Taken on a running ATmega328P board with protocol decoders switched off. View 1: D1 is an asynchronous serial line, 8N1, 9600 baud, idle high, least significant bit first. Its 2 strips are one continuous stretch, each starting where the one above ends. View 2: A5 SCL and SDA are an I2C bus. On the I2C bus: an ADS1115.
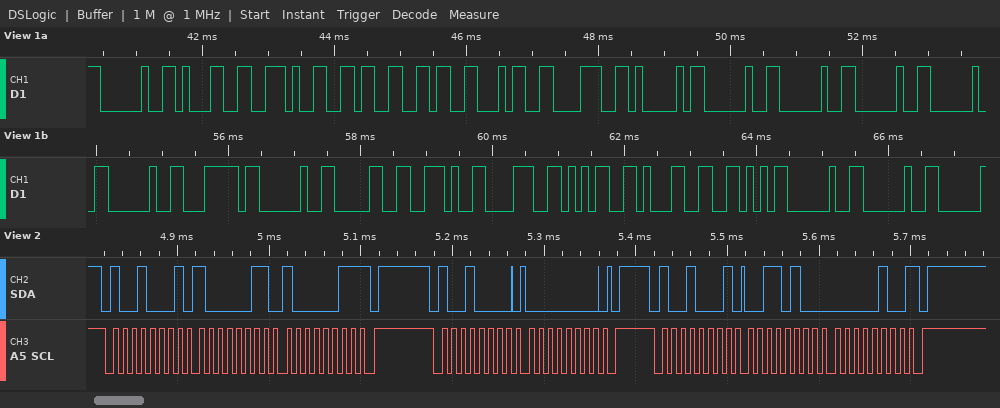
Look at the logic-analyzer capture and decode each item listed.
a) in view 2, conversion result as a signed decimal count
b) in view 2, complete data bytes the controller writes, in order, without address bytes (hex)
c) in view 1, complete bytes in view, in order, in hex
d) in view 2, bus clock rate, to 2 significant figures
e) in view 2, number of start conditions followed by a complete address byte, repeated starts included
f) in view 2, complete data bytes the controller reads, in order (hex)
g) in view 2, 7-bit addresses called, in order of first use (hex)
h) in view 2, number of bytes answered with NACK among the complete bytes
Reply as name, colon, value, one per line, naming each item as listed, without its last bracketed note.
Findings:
in view 2, conversion result as a signed decimal count: 13316
in view 2, complete data bytes the controller writes, in order, without address bytes: 00
in view 1, complete bytes in view, in order, in hex: 20 31 2E 36 36 34 38 41 20 20 20 20 20 7C 20 30 2E 38 35 31 56 20 20
in view 2, bus clock rate, to 2 significant figures: 100 kHz
in view 2, number of start conditions followed by a complete address byte, repeated starts included: 3
in view 2, complete data bytes the controller reads, in order: 83 83 34 04
in view 2, 7-bit addresses called, in order of first use: 0x48
in view 2, number of bytes answered with NACK among the complete bytes: 2
